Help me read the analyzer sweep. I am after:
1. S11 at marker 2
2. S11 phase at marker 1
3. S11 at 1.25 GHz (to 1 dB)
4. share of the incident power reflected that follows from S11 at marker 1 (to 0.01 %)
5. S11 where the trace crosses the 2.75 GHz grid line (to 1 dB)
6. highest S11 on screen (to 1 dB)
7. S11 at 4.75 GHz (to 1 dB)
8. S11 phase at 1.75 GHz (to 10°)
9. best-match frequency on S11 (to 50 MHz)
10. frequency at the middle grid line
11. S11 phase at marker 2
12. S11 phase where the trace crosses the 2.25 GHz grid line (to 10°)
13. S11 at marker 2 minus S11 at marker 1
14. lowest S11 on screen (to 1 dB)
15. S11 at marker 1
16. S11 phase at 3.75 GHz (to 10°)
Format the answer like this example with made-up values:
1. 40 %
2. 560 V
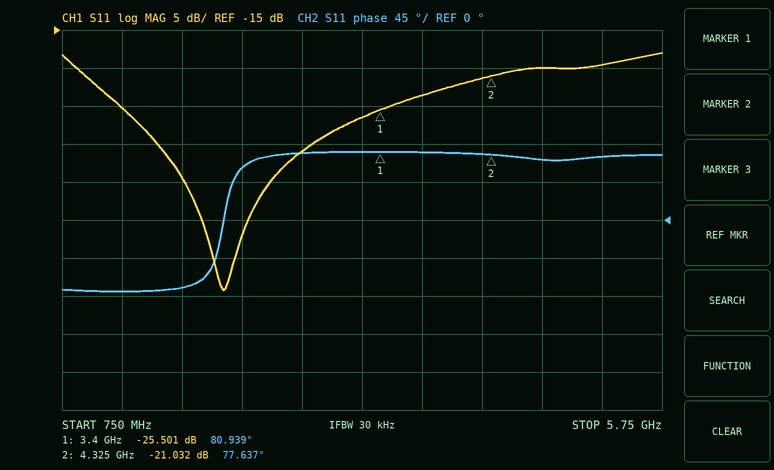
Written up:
1. -21.032 dB
2. 80.939°
3. -25 dB
4. 0.28 %
5. -31 dB
6. -18 dB
7. -20 dB
8. -80°
9. 2.10 GHz
10. 3.25 GHz
11. 77.637°
12. 60°
13. 4.469 dB
14. -49 dB
15. -25.501 dB
16. 80°
